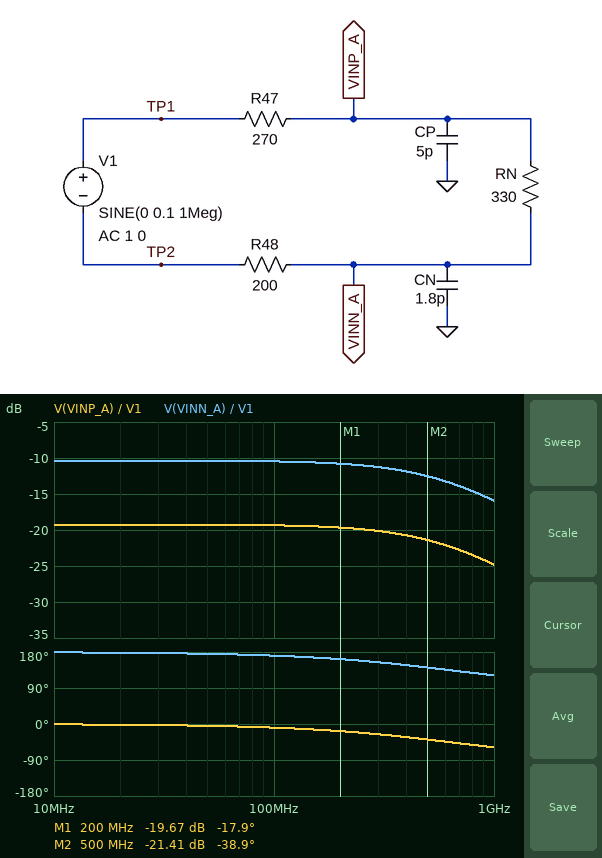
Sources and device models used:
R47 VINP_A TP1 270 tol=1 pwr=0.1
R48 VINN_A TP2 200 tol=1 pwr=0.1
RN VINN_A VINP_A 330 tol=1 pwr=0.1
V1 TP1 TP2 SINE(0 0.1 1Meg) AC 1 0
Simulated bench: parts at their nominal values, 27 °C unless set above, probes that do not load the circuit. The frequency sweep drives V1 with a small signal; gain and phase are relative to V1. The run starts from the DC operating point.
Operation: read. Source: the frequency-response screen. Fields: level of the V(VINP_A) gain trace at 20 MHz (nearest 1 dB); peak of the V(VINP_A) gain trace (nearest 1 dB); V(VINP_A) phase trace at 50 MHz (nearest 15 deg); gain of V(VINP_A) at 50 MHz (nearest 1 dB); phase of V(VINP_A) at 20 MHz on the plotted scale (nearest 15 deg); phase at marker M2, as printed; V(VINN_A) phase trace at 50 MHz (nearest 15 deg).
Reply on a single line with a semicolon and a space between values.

-19 dB; -19 dB; 0 deg; -19 dB; 0 deg; -38.9 deg; 180 deg
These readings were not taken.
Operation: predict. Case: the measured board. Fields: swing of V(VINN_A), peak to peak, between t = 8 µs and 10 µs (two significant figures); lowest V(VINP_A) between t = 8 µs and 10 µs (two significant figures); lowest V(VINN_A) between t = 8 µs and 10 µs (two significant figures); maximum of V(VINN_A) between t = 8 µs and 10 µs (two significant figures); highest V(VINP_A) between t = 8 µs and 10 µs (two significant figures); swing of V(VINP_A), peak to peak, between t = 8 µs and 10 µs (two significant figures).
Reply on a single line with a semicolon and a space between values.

61 mV; -11 mV; -30 mV; 30 mV; 11 mV; 22 mV
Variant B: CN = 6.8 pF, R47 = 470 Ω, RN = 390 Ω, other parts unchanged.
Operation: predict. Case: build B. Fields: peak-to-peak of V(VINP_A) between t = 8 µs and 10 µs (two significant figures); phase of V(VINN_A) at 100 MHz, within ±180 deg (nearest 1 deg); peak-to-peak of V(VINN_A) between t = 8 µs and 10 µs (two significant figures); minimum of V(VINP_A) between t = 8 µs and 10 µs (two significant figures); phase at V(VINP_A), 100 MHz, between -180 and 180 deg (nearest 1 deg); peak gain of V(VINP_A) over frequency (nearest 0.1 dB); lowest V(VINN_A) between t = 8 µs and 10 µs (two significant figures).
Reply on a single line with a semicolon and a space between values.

42 mV; 156 deg; 31 mV; -21 mV; -24 deg; -13.5 dB; -16 mV
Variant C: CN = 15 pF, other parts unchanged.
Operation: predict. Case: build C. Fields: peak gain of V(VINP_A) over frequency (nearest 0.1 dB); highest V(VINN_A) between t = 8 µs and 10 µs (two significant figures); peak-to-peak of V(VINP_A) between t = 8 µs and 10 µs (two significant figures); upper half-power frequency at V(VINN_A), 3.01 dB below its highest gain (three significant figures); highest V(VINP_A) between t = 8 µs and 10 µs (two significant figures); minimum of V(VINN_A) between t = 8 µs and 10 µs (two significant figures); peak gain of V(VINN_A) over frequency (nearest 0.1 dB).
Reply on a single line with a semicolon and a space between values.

-10.2 dB; 10 mV; 62 mV; 219 MHz; 31 mV; -10 mV; -19.7 dB
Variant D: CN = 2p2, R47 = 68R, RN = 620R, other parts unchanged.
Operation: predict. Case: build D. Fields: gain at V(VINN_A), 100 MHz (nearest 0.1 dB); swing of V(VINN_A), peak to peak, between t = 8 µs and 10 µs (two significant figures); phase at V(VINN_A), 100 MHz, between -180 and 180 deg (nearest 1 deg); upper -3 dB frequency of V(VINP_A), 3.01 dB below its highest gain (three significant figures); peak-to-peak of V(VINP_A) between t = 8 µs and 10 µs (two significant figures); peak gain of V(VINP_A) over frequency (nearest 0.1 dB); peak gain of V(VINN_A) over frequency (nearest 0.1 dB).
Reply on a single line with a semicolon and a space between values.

-6.4 dB; 97 mV; 170 deg; 557 MHz; 43 mV; -13.4 dB; -6.3 dB
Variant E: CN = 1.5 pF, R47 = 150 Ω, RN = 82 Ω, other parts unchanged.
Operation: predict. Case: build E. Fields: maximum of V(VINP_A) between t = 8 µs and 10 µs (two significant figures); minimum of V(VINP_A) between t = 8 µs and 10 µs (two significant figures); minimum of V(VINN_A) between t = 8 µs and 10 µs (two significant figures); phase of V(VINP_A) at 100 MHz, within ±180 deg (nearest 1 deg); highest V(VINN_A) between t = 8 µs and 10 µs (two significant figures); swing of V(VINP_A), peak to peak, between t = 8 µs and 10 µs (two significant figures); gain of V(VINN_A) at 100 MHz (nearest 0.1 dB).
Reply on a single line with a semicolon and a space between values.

4.4 mV; -4.4 mV; -15 mV; -3 deg; 15 mV; 8.8 mV; -16.7 dB
